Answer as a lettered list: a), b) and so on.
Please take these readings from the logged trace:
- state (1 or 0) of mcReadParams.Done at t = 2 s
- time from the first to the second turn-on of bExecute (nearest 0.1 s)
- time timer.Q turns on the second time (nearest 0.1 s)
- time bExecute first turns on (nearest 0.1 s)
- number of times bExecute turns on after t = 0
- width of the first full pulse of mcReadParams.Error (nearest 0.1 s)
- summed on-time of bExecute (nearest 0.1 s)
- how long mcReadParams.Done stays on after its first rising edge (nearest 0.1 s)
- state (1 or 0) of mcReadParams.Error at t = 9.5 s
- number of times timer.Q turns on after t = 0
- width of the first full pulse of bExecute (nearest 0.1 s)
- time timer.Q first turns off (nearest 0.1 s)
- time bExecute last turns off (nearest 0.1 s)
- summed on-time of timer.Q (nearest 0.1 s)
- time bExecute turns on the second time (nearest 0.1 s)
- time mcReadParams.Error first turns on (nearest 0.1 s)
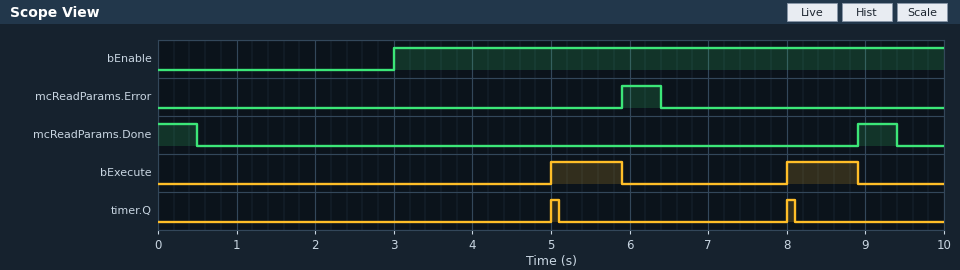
a) 0
b) 3.0 s
c) 8.0 s
d) 5.0 s
e) 2
f) 0.5 s
g) 1.8 s
h) 0.5 s
i) 0
j) 2
k) 0.9 s
l) 5.1 s
m) 8.9 s
n) 0.2 s
o) 8.0 s
p) 5.9 s
